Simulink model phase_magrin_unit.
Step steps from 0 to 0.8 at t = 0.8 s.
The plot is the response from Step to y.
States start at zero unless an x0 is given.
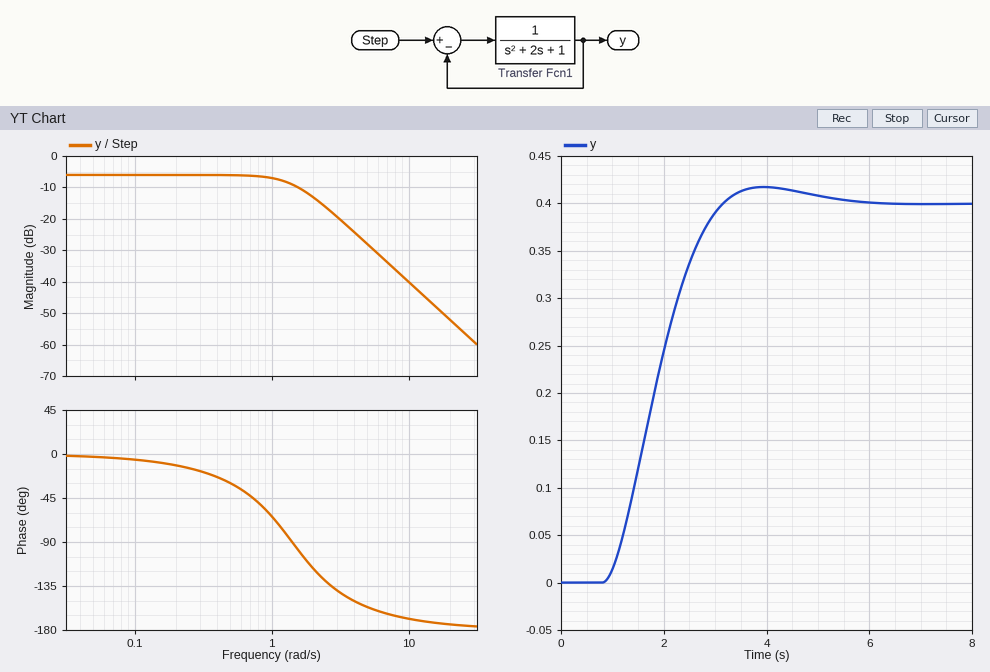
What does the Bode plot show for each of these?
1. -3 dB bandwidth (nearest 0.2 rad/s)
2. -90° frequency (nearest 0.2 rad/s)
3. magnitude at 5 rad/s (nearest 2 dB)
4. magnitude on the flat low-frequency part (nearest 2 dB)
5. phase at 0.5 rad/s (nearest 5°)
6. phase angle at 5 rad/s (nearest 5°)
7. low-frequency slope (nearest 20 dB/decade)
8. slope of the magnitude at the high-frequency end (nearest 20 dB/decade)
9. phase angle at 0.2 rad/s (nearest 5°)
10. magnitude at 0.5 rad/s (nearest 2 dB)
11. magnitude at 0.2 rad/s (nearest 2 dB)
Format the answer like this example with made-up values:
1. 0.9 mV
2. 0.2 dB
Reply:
1. 1.4 rad/s
2. 1.4 rad/s
3. -28 dB
4. -6 dB
5. -30°
6. -155°
7. 0 dB/decade
8. -40 dB/decade
9. -10°
10. -6 dB
11. -6 dB
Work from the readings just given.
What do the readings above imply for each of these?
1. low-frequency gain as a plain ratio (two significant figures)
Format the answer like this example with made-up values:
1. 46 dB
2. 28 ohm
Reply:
1. 0.50
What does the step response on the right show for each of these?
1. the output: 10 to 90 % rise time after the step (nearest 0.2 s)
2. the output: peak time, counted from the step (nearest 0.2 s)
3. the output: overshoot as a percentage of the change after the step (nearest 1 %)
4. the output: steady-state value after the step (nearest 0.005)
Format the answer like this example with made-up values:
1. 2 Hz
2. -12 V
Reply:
1. 1.6 s
2. 3.2 s
3. 4 %
4. 0.400
